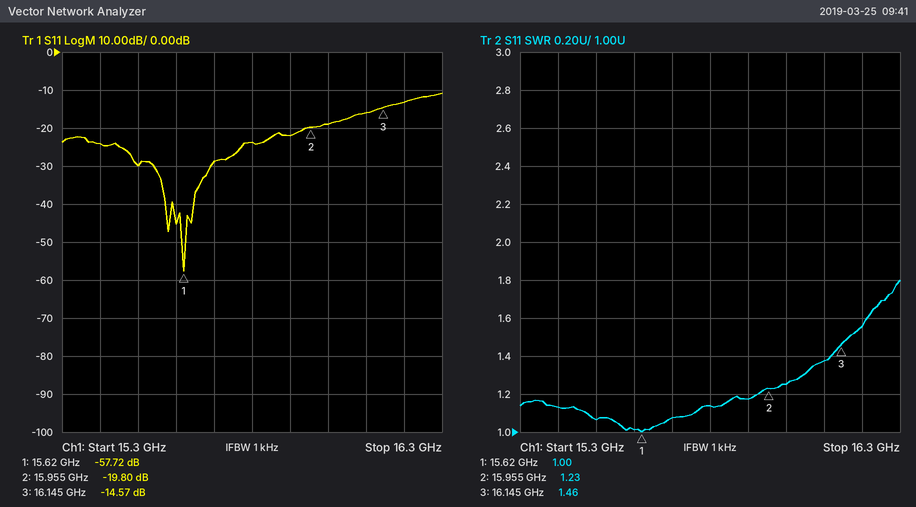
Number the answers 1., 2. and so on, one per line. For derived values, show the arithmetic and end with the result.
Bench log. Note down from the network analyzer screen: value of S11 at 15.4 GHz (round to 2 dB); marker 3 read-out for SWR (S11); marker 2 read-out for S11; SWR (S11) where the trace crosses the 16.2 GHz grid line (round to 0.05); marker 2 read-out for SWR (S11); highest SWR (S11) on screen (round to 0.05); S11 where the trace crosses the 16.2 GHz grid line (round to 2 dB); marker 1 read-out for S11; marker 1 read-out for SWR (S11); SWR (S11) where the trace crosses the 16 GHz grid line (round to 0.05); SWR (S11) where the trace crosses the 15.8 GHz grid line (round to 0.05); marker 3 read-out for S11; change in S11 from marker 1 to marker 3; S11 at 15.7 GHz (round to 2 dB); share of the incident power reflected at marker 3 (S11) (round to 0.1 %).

1. -24 dB
2. 1.46
3. -19.80 dB
4. 1.55
5. 1.23
6. 1.80
7. -14 dB
8. -57.72 dB
9. 1.00
10. 1.25
11. 1.15
12. -14.57 dB
13. -14.57 − (-57.72) = 43.15 dB
14. -28 dB
15. 10^(-14.57/10) ≈ 3.5 %
